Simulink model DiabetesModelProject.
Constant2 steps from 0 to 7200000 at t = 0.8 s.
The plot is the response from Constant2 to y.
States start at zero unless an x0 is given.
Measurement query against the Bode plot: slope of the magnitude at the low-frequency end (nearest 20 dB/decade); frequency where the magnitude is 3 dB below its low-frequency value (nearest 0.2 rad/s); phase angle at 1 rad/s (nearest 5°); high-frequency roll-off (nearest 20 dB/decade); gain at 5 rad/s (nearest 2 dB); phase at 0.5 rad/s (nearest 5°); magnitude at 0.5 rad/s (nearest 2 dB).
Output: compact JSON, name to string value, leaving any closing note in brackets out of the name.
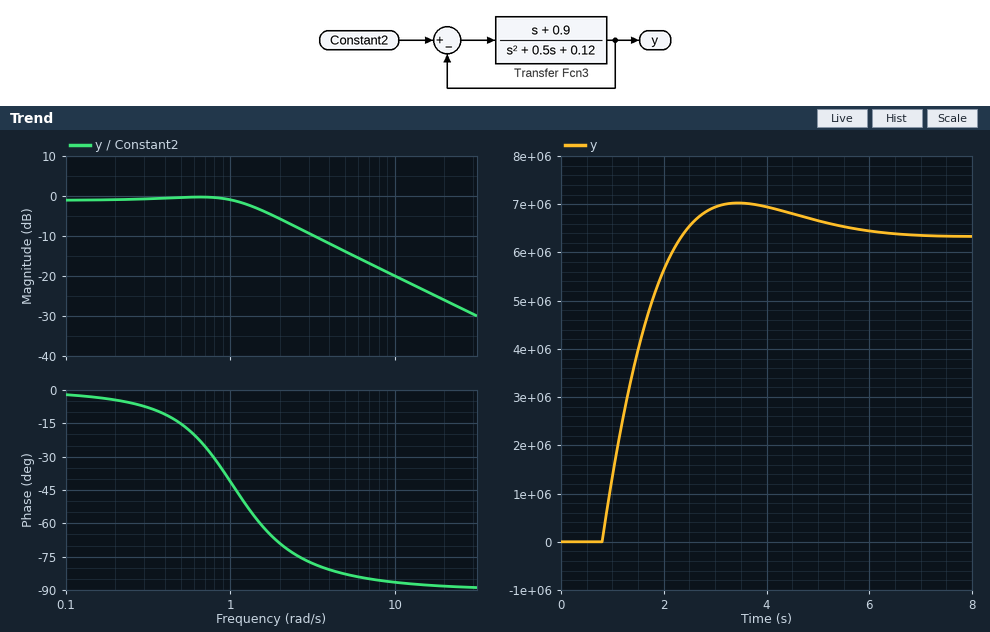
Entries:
{"slope of the magnitude at the low-frequency end": "0 dB/decade", "frequency where the magnitude is 3 dB below its low-frequency value": "1.6 rad/s", "phase angle at 1 rad/s": "-40°", "high-frequency roll-off": "-20 dB/decade", "gain at 5 rad/s": "-14 dB", "phase at 0.5 rad/s": "-15°", "magnitude at 0.5 rad/s": "0 dB"}
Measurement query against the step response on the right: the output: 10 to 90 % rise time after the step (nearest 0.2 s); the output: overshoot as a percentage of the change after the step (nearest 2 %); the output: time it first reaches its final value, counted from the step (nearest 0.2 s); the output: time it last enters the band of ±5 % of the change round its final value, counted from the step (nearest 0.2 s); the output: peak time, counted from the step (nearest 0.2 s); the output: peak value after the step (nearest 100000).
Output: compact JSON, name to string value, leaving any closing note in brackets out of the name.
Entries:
{"the output: 10 to 90 % rise time after the step": "1.2 s", "the output: overshoot as a percentage of the change after the step": "10 %", "the output: time it first reaches its final value, counted from the step": "1.6 s", "the output: time it last enters the band of ±5 % of the change round its final value, counted from the step": "4.2 s", "the output: peak time, counted from the step": "2.6 s", "the output: peak value after the step": "7000000"}
